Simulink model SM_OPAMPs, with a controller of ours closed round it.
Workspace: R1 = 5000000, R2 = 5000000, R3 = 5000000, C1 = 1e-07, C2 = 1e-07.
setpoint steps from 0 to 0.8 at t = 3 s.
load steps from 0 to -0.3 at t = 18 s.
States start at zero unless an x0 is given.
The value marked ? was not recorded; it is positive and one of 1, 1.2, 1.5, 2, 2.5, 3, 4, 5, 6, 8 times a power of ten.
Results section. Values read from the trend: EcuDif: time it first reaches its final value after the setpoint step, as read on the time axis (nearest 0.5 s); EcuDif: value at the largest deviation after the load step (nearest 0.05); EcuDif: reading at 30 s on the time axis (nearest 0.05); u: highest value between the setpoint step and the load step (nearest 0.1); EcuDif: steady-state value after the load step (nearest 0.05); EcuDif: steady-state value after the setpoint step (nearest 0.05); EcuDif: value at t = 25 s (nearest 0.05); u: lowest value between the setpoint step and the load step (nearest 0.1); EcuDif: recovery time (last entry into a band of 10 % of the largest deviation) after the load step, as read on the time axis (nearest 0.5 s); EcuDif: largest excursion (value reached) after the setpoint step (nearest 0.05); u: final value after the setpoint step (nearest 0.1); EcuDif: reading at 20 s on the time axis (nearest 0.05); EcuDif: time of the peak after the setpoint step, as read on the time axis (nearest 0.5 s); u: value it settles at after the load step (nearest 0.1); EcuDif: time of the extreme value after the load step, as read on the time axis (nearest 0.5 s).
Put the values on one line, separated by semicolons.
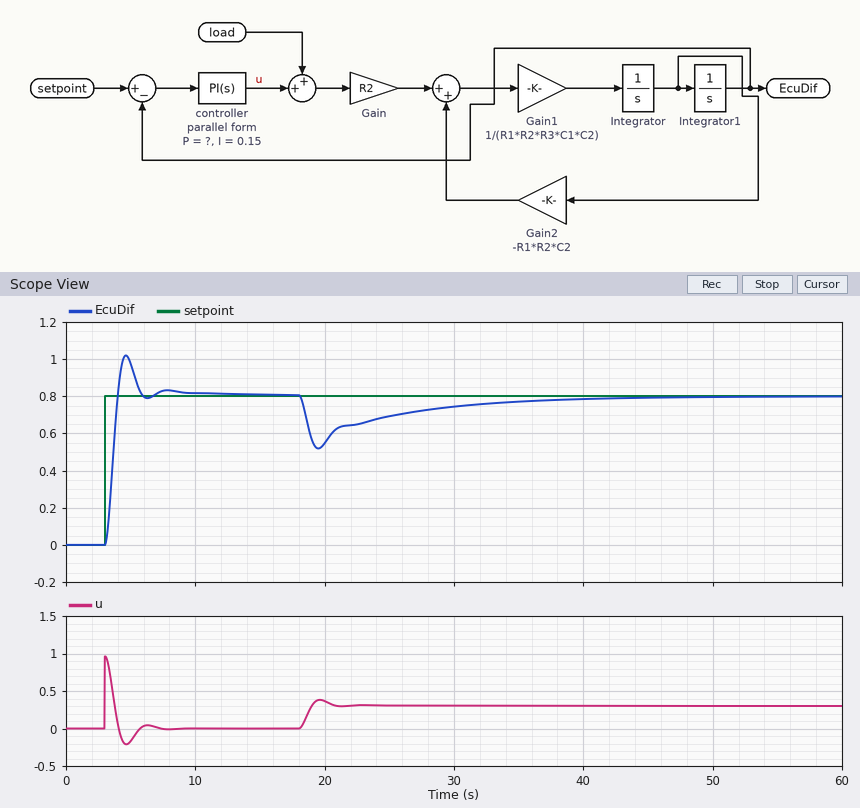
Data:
4.0 s; 0.50; 0.75; 1.0; 0.80; 0.80; 0.70; -0.2; 35.0 s; 1.00; 0.0; 0.55; 4.5 s; 0.3; 19.5 s
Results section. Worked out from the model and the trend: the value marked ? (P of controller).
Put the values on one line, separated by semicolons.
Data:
1.2
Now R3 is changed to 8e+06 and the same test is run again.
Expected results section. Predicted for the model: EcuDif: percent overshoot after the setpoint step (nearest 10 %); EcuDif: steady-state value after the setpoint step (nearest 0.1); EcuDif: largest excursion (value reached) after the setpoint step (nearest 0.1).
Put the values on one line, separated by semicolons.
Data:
40 %; 0.8; 1.1
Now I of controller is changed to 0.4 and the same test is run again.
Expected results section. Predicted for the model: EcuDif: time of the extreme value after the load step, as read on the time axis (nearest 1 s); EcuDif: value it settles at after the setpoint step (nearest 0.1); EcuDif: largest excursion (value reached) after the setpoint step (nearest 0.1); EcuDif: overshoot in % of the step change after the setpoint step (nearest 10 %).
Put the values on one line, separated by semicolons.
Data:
19 s; 0.8; 1.1; 40 %
